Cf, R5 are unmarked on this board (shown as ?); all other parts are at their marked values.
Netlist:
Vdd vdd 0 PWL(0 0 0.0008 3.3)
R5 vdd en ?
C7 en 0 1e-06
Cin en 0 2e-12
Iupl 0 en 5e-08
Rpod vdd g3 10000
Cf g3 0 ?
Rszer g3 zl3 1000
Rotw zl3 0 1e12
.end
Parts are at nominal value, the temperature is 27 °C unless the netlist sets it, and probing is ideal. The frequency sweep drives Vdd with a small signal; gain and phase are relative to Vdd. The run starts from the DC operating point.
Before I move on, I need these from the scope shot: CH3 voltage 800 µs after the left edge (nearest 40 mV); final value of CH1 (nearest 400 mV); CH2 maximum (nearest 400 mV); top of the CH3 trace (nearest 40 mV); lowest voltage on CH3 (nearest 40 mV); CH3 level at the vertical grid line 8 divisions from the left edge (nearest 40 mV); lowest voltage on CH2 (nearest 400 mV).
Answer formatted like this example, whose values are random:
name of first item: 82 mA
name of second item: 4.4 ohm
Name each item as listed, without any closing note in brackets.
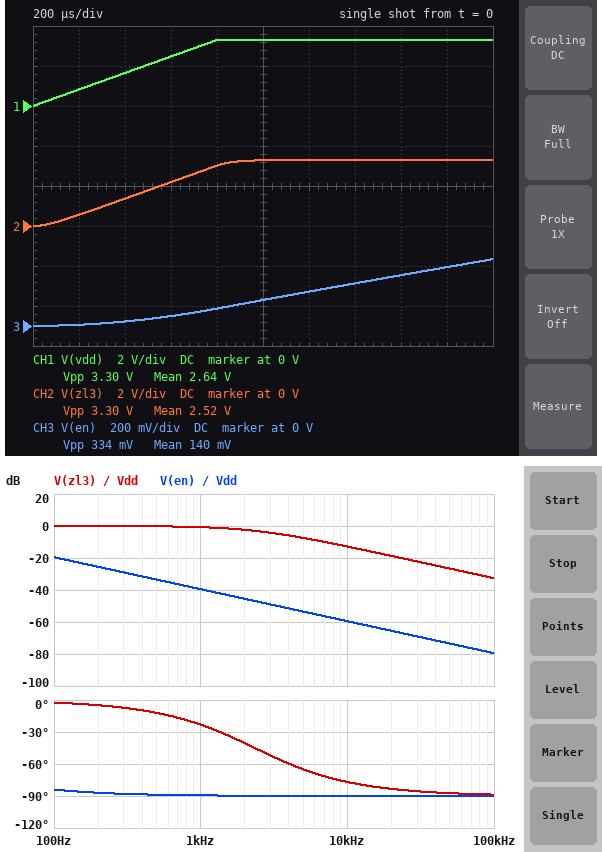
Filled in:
CH3 voltage 800 µs after the left edge: 80 mV
final value of CH1: 3.2 V
CH2 maximum: 3.2 V
top of the CH3 trace: 320 mV
lowest voltage on CH3: 0 V
CH3 level at the vertical grid line 8 divisions from the left edge: 240 mV
lowest voltage on CH2: 0 V
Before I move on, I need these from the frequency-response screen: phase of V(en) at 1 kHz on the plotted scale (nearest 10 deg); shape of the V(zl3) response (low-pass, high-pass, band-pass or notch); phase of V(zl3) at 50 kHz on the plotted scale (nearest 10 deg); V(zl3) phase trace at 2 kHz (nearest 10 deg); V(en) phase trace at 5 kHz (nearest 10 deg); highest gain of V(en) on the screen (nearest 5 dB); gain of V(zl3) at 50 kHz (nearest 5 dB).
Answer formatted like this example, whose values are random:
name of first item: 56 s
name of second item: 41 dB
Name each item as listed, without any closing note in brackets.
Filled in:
phase of V(en) at 1 kHz on the plotted scale: -90 deg
shape of the V(zl3) response: low-pass
phase of V(zl3) at 50 kHz on the plotted scale: -90 deg
V(zl3) phase trace at 2 kHz: -40 deg
V(en) phase trace at 5 kHz: -90 deg
highest gain of V(en) on the screen: -20 dB
gain of V(zl3) at 50 kHz: -25 dB
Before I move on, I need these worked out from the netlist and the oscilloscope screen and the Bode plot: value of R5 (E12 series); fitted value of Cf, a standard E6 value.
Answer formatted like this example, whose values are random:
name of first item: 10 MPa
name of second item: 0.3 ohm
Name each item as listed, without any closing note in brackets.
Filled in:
value of R5: 15 kΩ
fitted value of Cf, a standard E6 value: 6.8 nF
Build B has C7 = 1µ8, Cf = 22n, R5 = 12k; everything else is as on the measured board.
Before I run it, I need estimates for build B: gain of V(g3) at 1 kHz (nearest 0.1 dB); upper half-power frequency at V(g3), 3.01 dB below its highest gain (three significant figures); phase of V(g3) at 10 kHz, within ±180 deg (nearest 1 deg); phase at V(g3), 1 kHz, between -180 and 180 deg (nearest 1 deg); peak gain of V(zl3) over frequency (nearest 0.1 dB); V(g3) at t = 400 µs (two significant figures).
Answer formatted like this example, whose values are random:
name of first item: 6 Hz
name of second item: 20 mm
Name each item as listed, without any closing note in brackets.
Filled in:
gain of V(g3) at 1 kHz: -4.6 dB
upper half-power frequency at V(g3), 3.01 dB below its highest gain: 723 Hz
phase of V(g3) at 10 kHz, within ±180 deg: -86 deg
phase at V(g3), 1 kHz, between -180 and 180 deg: -54 deg
peak gain of V(zl3) over frequency: 0 dB
V(g3) at t = 400 µs: 890 mV
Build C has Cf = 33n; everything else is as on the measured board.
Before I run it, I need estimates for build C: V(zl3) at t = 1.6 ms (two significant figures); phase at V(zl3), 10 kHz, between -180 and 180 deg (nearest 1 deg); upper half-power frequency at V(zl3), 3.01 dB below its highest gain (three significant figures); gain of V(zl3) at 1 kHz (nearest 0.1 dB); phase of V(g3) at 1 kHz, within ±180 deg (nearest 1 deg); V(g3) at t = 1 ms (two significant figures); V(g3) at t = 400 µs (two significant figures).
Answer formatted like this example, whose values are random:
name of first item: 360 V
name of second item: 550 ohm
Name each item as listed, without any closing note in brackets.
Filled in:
V(zl3) at t = 1.6 ms: 3.2 V
phase at V(zl3), 10 kHz, between -180 and 180 deg: -87 deg
upper half-power frequency at V(zl3), 3.01 dB below its highest gain: 482 Hz
gain of V(zl3) at 1 kHz: -7.2 dB
phase of V(g3) at 1 kHz, within ±180 deg: -64 deg
V(g3) at t = 1 ms: 2.6 V
V(g3) at t = 400 µs: 690 mV
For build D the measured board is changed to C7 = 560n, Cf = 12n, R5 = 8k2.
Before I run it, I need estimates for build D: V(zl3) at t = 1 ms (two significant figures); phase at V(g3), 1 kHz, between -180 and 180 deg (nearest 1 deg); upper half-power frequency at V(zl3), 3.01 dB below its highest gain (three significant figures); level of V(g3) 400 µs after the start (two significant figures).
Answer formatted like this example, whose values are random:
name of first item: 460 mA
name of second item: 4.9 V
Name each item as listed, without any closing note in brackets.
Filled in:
V(zl3) at t = 1 ms: 3.2 V
phase at V(g3), 1 kHz, between -180 and 180 deg: -37 deg
upper half-power frequency at V(zl3), 3.01 dB below its highest gain: 1.33 kHz
level of V(g3) 400 µs after the start: 1.2 V
